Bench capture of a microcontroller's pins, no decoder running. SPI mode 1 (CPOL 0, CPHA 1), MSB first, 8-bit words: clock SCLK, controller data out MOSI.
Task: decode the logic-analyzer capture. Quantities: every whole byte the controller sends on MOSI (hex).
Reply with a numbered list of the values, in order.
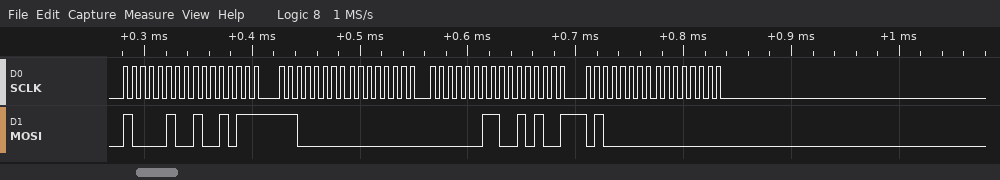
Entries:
1. 0x84 0x97 0xC0 0x00 0x03 0x29 0x40 0x00
